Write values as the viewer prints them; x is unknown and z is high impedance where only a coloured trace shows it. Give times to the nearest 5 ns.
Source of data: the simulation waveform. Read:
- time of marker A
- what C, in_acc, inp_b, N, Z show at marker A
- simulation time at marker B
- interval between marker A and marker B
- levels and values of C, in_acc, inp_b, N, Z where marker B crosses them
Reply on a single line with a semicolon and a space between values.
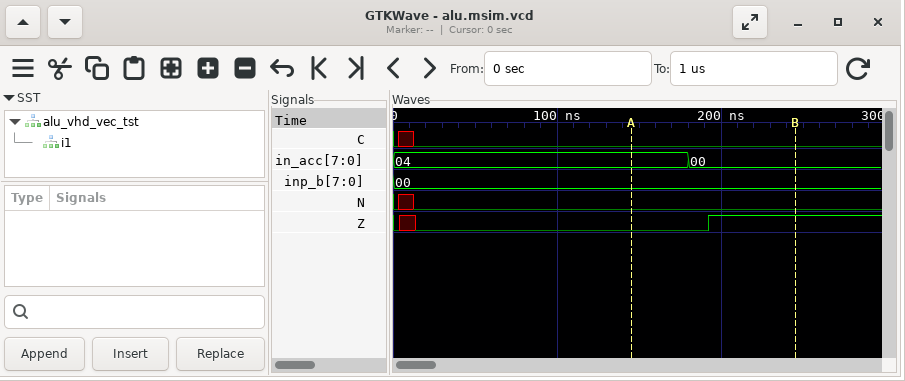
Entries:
145 ns; C=0, in_acc=04, inp_b=00, N=0, Z=0; 245 ns; 100 ns; C=0, in_acc=00, inp_b=00, N=0, Z=1
